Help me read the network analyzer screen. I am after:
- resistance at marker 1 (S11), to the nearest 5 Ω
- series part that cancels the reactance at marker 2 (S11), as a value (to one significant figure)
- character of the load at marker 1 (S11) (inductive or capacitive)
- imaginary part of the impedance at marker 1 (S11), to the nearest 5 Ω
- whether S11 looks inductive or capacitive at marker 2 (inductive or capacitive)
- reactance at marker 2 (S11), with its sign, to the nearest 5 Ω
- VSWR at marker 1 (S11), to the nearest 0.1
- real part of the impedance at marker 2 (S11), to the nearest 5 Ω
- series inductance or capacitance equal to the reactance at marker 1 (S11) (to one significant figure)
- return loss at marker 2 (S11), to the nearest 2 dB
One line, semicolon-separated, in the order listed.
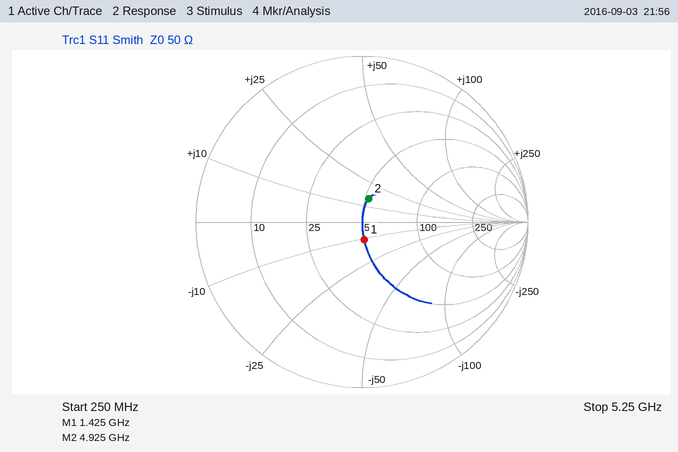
50 Ω; 2 pF; capacitive; -10 Ω; inductive; +15 Ω; 1.2; 50 Ω; 10 pF; 16 dB
